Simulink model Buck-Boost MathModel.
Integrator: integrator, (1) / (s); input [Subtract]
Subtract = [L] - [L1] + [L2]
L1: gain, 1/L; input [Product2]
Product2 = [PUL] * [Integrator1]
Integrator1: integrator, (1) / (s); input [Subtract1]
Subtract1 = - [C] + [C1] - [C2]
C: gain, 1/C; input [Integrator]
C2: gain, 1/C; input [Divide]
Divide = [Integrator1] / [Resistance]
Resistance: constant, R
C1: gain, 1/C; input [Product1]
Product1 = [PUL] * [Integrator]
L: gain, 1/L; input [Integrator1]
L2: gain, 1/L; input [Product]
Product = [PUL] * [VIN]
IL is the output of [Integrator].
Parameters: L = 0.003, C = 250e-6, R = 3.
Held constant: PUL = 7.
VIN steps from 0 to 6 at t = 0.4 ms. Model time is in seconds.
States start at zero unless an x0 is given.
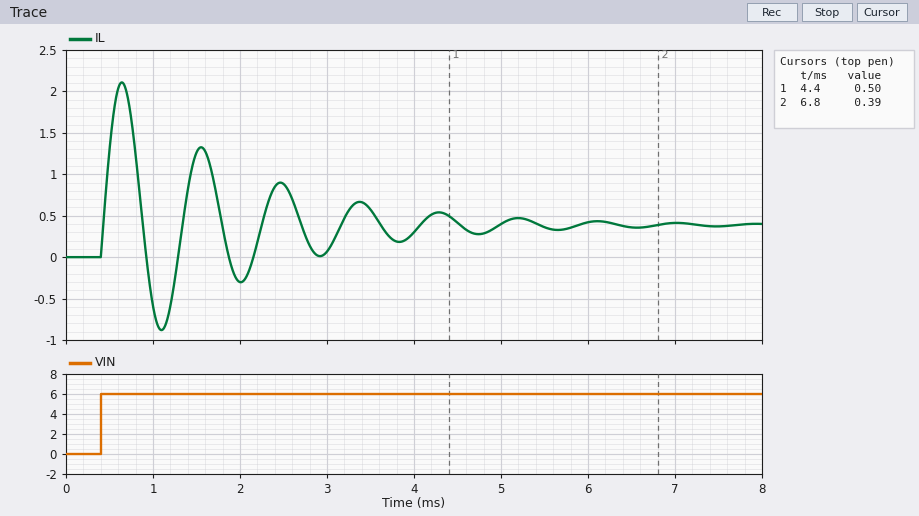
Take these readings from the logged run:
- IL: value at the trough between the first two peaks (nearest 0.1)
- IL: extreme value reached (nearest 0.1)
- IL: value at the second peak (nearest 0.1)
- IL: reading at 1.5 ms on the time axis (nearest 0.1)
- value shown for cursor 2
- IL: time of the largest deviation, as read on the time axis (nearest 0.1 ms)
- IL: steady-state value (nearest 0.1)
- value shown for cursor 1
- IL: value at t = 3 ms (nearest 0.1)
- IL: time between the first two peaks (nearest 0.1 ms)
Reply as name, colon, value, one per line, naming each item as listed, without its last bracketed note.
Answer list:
IL: value at the trough between the first two peaks: -0.9
IL: extreme value reached: 2.1
IL: value at the second peak: 1.3
IL: reading at 1.5 ms on the time axis: 1.3
value shown for cursor 2: 0.39
IL: time of the largest deviation, as read on the time axis: 0.6 ms
IL: steady-state value: 0.4
value shown for cursor 1: 0.50
IL: value at t = 3 ms: 0.1
IL: time between the first two peaks: 0.9 ms
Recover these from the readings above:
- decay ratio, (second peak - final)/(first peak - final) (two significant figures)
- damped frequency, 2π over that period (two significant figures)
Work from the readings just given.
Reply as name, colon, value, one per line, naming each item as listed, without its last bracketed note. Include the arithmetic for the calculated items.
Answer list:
decay ratio, (second peak - final)/(first peak - final): (1.3 - 0.4) / (2.1 - 0.4) = 0.53
damped frequency, 2π over that period: 2π / 0.9 = 7.0 rad/ms
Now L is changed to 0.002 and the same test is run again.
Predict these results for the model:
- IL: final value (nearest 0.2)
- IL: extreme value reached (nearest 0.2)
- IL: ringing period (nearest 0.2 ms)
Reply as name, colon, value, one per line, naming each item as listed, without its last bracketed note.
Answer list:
IL: final value: 0.4
IL: extreme value reached: 2.6
IL: ringing period: 0.8 ms
